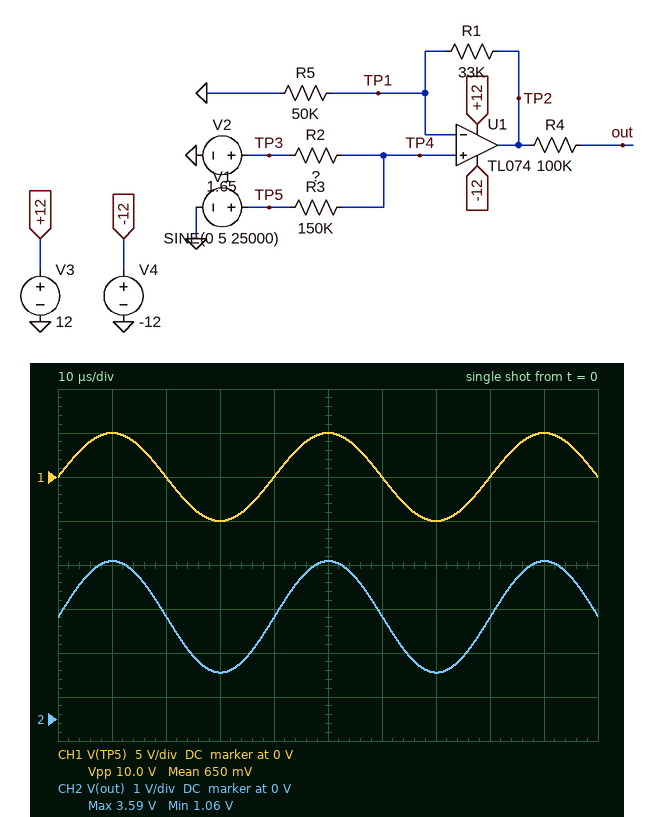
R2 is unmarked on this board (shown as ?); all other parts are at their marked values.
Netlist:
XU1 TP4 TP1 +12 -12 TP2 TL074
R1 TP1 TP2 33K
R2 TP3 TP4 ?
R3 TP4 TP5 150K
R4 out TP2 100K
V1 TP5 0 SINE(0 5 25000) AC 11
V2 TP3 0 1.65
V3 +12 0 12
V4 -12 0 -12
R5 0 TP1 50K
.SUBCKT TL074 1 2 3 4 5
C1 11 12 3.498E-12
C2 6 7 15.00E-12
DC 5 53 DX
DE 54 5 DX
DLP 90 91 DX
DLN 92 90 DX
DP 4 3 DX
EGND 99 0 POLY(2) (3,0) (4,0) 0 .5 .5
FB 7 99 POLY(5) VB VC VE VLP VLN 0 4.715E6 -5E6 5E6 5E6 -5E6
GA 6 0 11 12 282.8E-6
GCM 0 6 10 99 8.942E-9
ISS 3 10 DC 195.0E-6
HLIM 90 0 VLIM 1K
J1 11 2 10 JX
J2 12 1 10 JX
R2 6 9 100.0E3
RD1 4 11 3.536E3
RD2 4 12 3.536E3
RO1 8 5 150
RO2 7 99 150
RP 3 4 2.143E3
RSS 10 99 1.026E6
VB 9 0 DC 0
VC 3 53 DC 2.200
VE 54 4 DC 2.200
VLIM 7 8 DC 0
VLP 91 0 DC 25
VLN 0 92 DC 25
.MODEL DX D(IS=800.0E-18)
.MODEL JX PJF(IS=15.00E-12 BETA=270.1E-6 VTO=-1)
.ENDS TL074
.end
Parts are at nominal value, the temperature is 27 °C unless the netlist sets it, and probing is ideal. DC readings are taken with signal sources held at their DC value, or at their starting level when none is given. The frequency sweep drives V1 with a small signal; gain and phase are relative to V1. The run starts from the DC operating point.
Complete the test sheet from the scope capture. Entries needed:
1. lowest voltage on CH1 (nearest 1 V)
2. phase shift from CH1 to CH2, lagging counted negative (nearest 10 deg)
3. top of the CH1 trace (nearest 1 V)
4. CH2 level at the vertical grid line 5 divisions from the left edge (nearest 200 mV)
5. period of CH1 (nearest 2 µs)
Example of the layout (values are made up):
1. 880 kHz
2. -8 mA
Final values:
1. -5 V
2. 0 deg
3. 5 V
4. 3.6 V
5. 40 µs
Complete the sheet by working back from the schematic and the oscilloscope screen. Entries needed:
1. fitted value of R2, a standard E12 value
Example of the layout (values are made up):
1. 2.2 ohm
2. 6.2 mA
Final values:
1. 27 kΩ
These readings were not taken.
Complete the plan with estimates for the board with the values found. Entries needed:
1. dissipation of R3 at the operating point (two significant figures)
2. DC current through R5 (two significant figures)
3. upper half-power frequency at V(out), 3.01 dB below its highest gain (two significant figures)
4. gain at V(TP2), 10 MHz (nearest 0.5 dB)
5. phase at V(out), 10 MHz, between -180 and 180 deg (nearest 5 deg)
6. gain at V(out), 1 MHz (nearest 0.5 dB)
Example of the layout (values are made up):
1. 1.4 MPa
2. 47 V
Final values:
1. 13 µW
2. 28 µA
3. 2.8 MHz
4. -30.0 dB
5. -145 deg
6. -12.5 dB
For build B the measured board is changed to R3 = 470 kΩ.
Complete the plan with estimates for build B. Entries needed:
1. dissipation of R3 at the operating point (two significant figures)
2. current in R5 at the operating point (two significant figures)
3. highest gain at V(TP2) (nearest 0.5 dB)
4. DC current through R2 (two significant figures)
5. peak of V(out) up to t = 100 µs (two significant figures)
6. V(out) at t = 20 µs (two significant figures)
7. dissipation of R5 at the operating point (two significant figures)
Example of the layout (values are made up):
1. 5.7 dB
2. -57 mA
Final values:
1. 5.2 µW
2. 31 µA
3. -21.0 dB
4. 3.3 µA
5. 3.0 V
6. 2.6 V
7. 49 µW
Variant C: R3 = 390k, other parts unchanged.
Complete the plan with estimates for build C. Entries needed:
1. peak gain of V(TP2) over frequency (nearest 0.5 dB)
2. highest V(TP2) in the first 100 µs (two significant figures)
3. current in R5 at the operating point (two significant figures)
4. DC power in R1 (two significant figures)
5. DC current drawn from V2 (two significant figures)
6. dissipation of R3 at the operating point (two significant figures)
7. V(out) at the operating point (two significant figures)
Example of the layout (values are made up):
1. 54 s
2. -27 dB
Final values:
1. -19.5 dB
2. 3.1 V
3. 31 µA
4. 31 µW
5. 4.0 µA
6. 6.1 µW
7. 2.6 V
